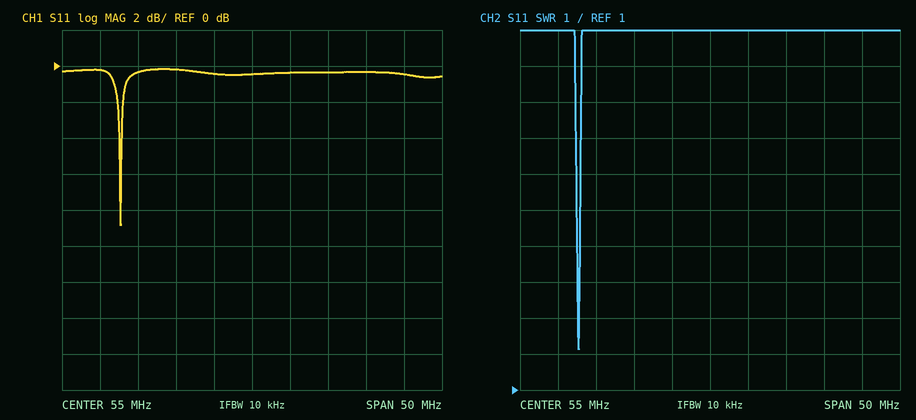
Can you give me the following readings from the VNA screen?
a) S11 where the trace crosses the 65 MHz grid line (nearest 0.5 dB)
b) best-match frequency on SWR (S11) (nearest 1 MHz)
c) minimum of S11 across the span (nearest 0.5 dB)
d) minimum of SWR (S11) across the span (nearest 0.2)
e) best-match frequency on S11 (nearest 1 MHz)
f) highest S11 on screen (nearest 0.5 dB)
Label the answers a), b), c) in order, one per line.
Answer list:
a) -0.5 dB
b) 38 MHz
c) -9.0 dB
d) 2.2
e) 38 MHz
f) 0.0 dB
